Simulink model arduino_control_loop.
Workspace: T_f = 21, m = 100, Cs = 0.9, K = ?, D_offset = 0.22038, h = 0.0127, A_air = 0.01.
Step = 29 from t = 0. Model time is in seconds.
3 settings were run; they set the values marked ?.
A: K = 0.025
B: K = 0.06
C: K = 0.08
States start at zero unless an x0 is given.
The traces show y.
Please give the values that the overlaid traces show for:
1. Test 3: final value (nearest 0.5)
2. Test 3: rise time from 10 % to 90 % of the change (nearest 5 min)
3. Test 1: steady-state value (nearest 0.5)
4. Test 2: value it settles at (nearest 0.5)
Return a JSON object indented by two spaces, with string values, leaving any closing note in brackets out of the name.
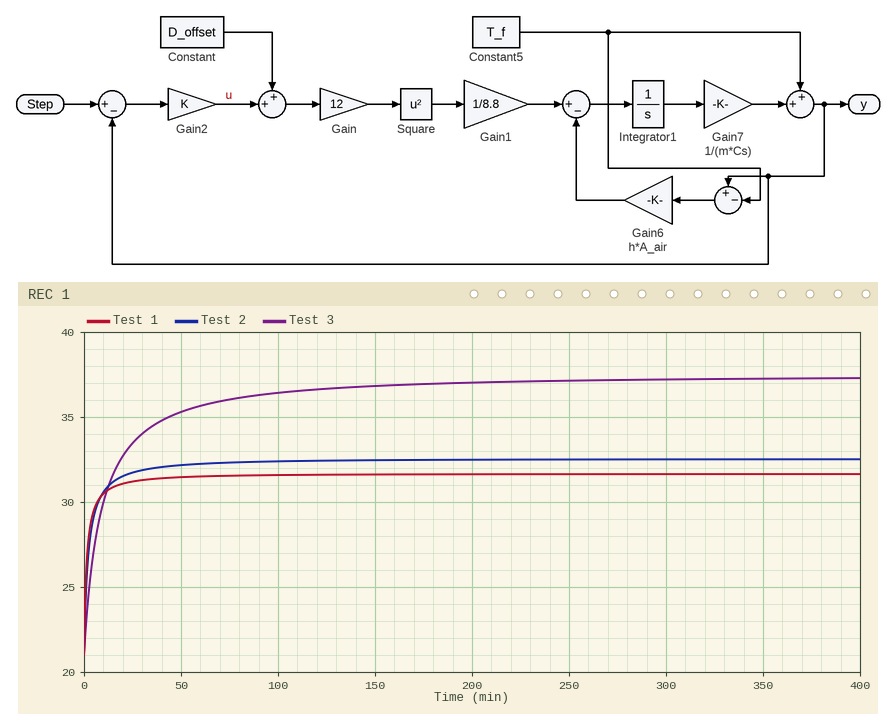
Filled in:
{
  "Test 3: final value": "37.5",
  "Test 3: rise time from 10 % to 90 % of the change": "60 min",
  "Test 1: steady-state value": "31.5",
  "Test 2: value it settles at": "32.5"
}
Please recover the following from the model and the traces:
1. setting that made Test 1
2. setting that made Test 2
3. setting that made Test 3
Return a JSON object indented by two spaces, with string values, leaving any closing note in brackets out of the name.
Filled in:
{
  "setting that made Test 1": "C",
  "setting that made Test 2": "B",
  "setting that made Test 3": "A"
}
